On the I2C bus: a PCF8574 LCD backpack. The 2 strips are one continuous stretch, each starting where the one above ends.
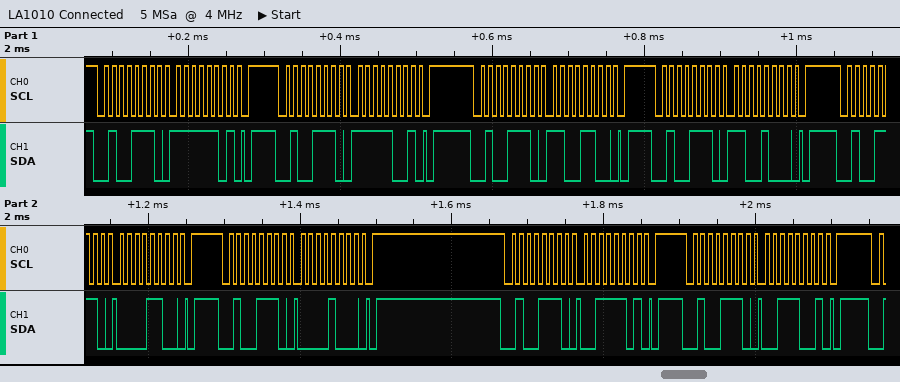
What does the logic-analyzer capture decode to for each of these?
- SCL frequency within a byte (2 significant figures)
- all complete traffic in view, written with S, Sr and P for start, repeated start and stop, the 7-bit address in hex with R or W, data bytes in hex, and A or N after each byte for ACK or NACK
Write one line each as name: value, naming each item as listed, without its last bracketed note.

SCL frequency within a byte: 100 kHz
all complete traffic in view, written with S, Sr and P for start, repeated start and stop, the 7-bit address in hex with R or W, data bytes in hex, and A or N after each byte for ACK or NACK: S 27W A FD A P S 27W A F9 A P S 27W A CC A P S 27W A C8 A P S 27W A 0C A P S 27W A 08 A P S 27W A 3D A P S 27W A 39 A P
